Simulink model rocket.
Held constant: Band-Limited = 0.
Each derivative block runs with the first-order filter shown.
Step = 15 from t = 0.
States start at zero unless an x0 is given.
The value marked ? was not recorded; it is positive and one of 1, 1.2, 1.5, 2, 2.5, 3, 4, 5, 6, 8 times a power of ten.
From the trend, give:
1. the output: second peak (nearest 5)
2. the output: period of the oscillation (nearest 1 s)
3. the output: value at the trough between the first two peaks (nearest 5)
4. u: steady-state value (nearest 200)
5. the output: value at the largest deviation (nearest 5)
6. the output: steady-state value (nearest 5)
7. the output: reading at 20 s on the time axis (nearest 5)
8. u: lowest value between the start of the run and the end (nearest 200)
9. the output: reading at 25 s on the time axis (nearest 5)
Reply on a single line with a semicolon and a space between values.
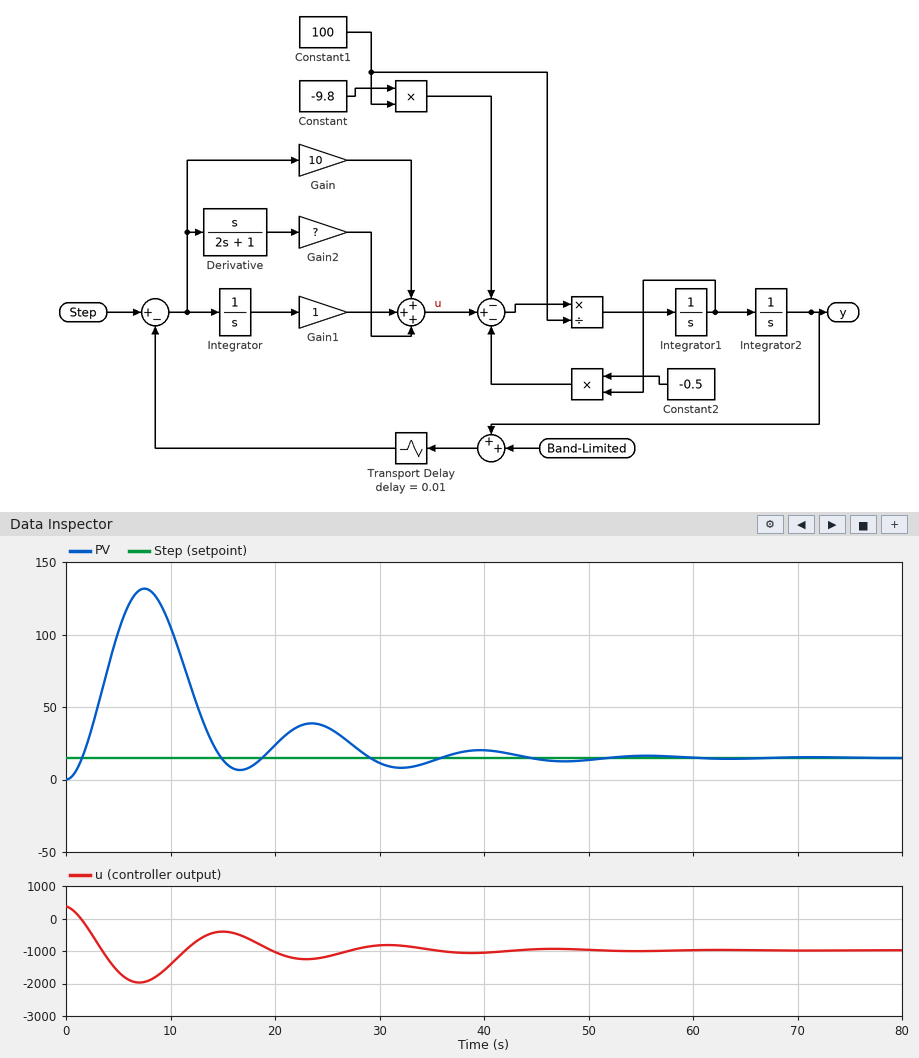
40; 16 s; 5; -1000; 130; 15; 25; -2000; 35
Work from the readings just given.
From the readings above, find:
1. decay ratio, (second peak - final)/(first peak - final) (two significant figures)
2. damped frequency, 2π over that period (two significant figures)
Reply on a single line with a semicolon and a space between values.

0.22; 0.39 rad/s
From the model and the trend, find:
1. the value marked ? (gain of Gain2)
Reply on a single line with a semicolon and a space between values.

30
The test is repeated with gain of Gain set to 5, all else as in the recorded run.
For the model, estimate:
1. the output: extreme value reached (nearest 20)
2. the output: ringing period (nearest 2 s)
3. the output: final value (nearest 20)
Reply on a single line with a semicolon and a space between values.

180; 26 s; 20
